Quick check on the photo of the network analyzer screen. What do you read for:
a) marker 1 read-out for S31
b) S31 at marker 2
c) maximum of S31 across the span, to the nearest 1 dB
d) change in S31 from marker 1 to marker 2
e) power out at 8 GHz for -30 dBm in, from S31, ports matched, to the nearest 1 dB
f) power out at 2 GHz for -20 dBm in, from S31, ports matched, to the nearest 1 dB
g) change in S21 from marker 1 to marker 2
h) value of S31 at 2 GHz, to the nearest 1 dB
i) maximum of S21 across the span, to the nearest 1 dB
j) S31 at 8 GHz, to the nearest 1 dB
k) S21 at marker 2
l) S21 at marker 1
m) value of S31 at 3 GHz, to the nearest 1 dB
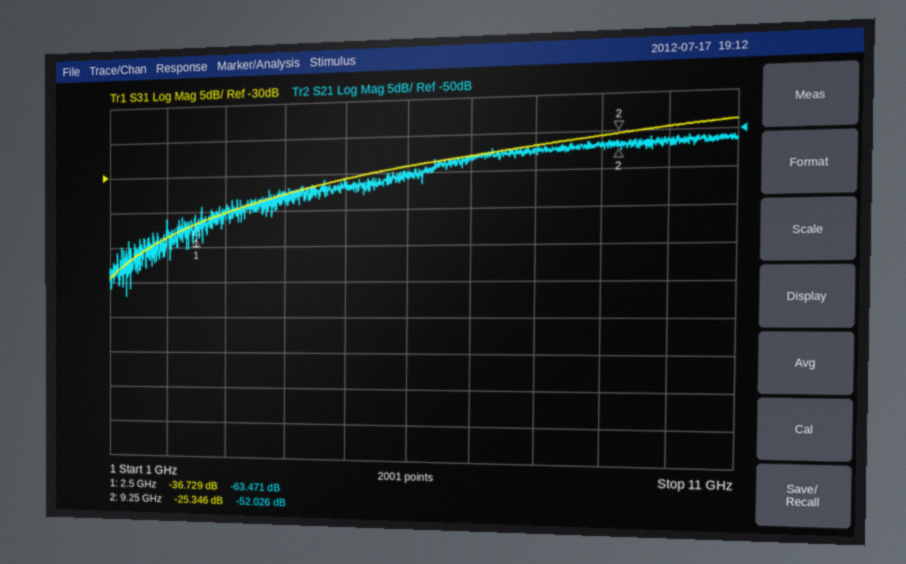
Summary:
-36.729 dB
-25.346 dB
-24 dB
11.383 dB
-57 dBm
-59 dBm
11.445 dB
-39 dB
-51 dB
-27 dB
-52.026 dB
-63.471 dB
-35 dB
